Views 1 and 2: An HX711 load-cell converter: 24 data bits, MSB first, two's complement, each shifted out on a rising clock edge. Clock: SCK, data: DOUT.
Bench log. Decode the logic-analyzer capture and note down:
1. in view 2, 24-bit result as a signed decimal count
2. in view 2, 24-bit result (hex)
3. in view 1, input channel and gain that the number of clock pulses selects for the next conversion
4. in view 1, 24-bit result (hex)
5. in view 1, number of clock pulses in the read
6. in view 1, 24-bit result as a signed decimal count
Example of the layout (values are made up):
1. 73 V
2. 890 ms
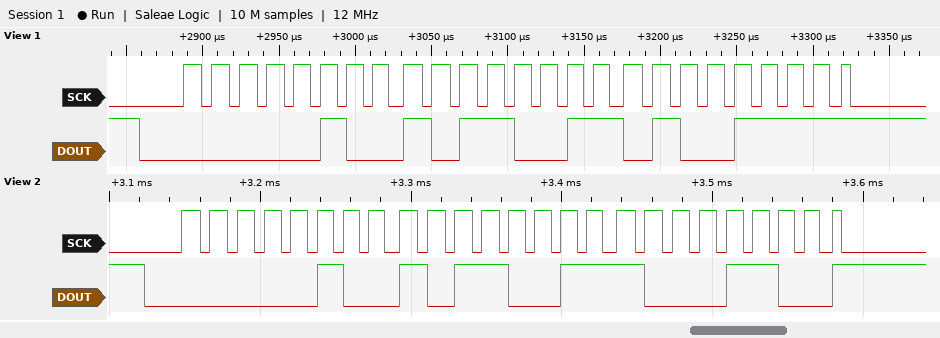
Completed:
1. 308108
2. 0x04B38C
3. channel A, gain 128
4. 0x04B34F
5. 25
6. 308047
